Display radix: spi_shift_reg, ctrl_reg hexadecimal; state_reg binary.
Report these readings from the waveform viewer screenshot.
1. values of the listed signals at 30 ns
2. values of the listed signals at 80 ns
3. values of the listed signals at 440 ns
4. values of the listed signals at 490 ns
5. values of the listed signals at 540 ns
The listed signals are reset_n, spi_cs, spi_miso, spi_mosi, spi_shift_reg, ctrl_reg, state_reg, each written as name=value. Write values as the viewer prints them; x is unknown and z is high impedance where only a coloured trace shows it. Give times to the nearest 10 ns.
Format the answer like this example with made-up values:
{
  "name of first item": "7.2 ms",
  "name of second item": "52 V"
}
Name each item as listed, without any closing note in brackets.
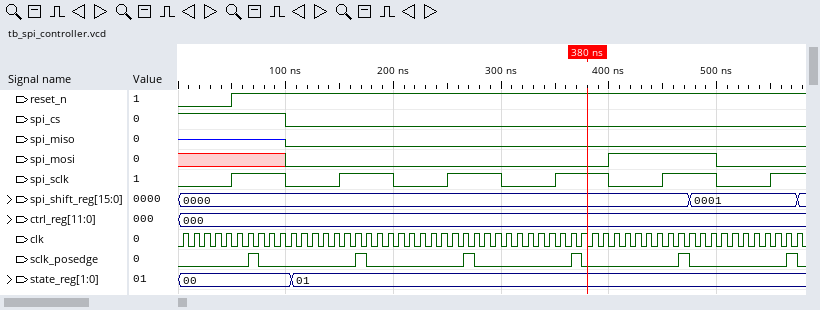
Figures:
{
  "values of the listed signals at 30 ns": "reset_n=0, spi_cs=1, spi_miso=z, spi_mosi=x, spi_shift_reg=0000, ctrl_reg=000, state_reg=00",
  "values of the listed signals at 80 ns": "reset_n=1, spi_cs=1, spi_miso=z, spi_mosi=x, spi_shift_reg=0000, ctrl_reg=000, state_reg=00",
  "values of the listed signals at 440 ns": "reset_n=1, spi_cs=0, spi_miso=0, spi_mosi=1, spi_shift_reg=0000, ctrl_reg=000, state_reg=01",
  "values of the listed signals at 490 ns": "reset_n=1, spi_cs=0, spi_miso=0, spi_mosi=1, spi_shift_reg=0001, ctrl_reg=000, state_reg=01",
  "values of the listed signals at 540 ns": "reset_n=1, spi_cs=0, spi_miso=0, spi_mosi=0, spi_shift_reg=0001, ctrl_reg=000, state_reg=01"
}
